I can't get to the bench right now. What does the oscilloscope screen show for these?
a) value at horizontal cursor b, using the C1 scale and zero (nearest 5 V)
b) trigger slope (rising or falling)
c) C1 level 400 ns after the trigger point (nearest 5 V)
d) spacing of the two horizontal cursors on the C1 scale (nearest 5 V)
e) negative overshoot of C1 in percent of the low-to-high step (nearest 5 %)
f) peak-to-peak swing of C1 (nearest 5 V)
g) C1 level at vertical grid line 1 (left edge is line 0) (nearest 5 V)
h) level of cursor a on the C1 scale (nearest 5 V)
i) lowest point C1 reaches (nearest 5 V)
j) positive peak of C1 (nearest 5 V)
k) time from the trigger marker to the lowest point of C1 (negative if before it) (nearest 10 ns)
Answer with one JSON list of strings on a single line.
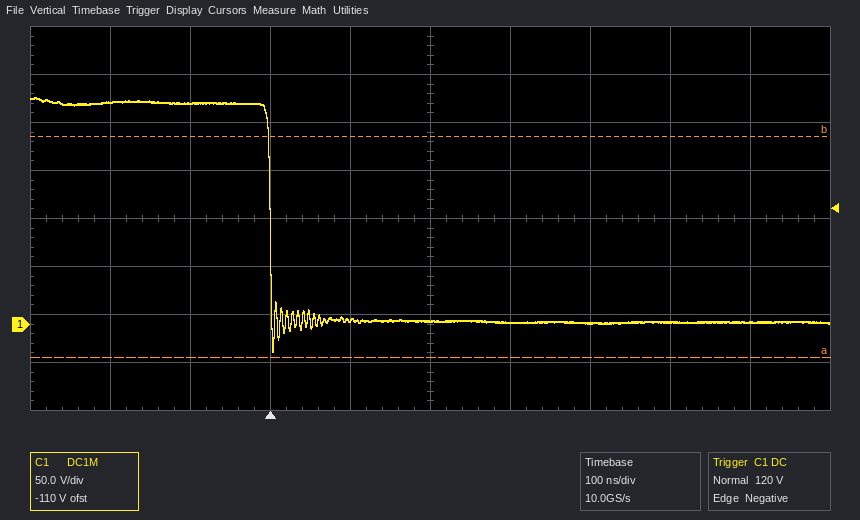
["195 V", "falling", "0 V", "230 V", "15 %", "265 V", "230 V", "-35 V", "-30 V", "235 V", "0 ns"]
